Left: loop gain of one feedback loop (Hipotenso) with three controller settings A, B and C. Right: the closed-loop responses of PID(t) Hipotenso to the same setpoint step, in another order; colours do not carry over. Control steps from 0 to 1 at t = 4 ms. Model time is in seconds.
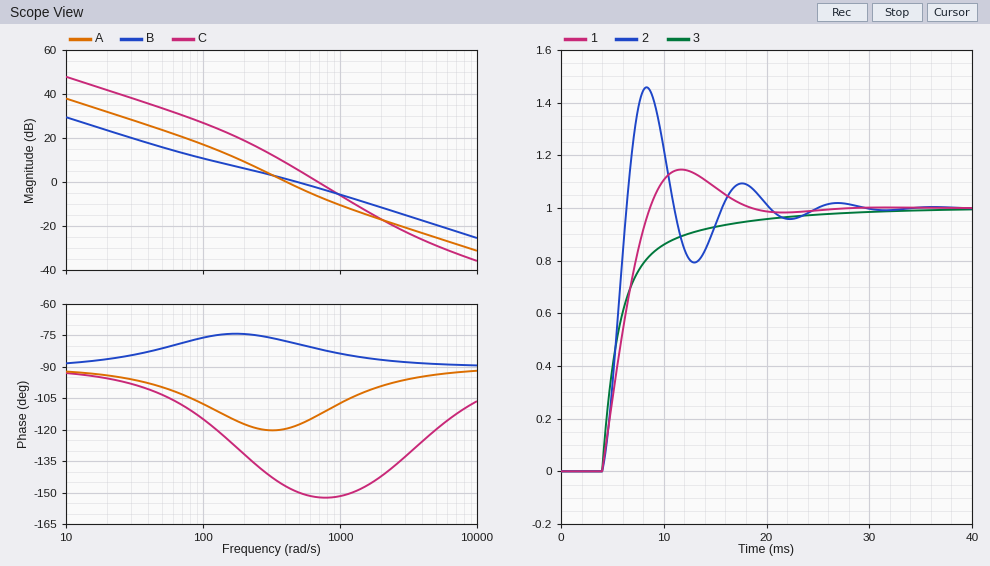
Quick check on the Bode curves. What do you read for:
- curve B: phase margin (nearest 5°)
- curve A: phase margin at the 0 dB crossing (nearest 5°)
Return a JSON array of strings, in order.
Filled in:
["100°", "60°"]
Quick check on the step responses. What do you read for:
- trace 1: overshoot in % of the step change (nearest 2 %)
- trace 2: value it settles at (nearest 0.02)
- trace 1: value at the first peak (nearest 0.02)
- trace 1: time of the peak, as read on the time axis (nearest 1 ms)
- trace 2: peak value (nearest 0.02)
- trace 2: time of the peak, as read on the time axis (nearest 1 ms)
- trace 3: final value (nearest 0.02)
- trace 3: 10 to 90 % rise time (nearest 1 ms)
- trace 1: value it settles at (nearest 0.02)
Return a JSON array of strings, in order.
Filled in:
["14 %", "1.00", "1.14", "12 ms", "1.46", "8 ms", "1.00", "8 ms", "1.00"]
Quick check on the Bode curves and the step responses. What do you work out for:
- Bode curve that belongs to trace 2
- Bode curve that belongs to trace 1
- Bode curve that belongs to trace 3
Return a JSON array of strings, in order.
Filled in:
["C", "A", "B"]
